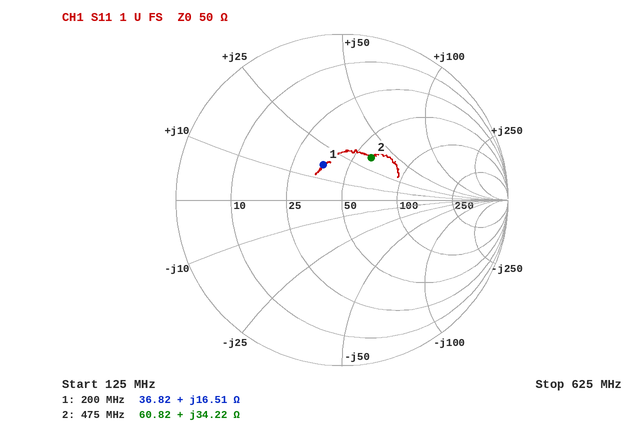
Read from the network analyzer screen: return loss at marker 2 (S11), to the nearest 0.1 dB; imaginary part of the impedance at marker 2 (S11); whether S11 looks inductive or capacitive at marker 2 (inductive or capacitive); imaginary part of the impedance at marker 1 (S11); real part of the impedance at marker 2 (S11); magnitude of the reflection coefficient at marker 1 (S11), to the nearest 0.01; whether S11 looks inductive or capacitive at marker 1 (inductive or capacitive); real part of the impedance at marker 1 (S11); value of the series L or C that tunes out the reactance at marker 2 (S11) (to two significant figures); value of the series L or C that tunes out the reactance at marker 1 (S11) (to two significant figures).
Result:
10.2 dB
+34.22 Ω
inductive
+16.51 Ω
60.82 Ω
0.24
inductive
36.82 Ω
9.8 pF
48 pF
